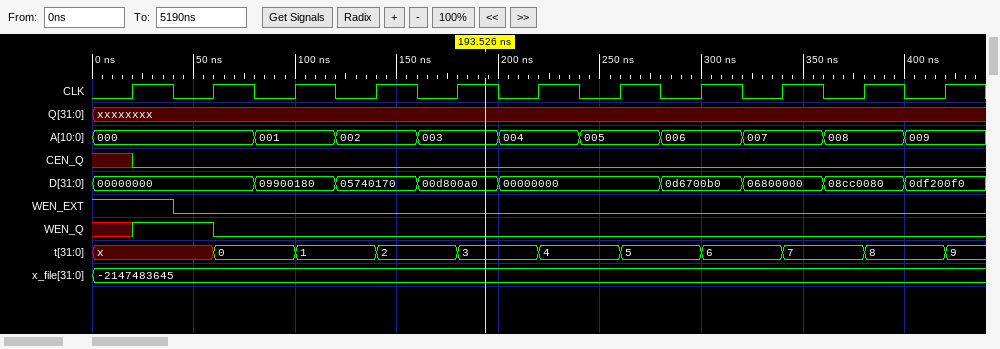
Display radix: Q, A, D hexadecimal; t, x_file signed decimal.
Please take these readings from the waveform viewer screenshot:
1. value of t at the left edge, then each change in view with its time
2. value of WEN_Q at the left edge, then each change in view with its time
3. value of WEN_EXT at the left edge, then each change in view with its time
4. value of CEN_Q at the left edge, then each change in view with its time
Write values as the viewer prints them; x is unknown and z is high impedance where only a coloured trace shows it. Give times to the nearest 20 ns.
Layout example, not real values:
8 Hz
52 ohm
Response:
x, 0 at 60 ns, 1 at 100 ns, 2 at 140 ns, 3 at 180 ns, 4 at 220 ns, 5 at 260 ns, 6 at 300 ns, 7 at 340 ns, 8 at 380 ns, 9 at 420 ns
x, 1 at 20 ns, 0 at 60 ns
1, 0 at 40 ns
x, 0 at 20 ns
